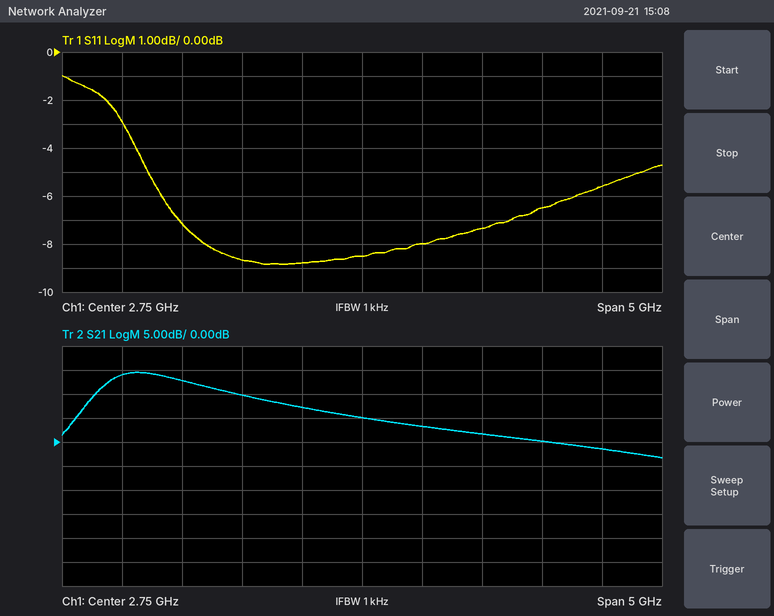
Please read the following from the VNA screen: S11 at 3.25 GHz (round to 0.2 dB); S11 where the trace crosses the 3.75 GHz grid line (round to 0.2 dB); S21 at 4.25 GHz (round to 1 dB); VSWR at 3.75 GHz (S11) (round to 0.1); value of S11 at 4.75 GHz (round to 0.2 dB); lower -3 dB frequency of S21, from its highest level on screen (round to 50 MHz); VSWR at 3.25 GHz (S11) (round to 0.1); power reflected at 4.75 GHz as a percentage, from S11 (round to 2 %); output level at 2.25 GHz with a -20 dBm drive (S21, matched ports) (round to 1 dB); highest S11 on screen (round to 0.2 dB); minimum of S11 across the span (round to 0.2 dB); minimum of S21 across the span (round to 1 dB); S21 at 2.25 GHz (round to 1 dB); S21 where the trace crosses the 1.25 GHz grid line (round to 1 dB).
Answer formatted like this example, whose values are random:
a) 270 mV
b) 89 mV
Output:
a) -8.0 dB
b) -7.4 dB
c) 0 dB
d) 2.5
e) -5.6 dB
f) 600 MHz
g) 2.3
h) 28 %
i) -13 dBm
j) -1.0 dB
k) -8.8 dB
l) -3 dB
m) 7 dB
n) 13 dB
